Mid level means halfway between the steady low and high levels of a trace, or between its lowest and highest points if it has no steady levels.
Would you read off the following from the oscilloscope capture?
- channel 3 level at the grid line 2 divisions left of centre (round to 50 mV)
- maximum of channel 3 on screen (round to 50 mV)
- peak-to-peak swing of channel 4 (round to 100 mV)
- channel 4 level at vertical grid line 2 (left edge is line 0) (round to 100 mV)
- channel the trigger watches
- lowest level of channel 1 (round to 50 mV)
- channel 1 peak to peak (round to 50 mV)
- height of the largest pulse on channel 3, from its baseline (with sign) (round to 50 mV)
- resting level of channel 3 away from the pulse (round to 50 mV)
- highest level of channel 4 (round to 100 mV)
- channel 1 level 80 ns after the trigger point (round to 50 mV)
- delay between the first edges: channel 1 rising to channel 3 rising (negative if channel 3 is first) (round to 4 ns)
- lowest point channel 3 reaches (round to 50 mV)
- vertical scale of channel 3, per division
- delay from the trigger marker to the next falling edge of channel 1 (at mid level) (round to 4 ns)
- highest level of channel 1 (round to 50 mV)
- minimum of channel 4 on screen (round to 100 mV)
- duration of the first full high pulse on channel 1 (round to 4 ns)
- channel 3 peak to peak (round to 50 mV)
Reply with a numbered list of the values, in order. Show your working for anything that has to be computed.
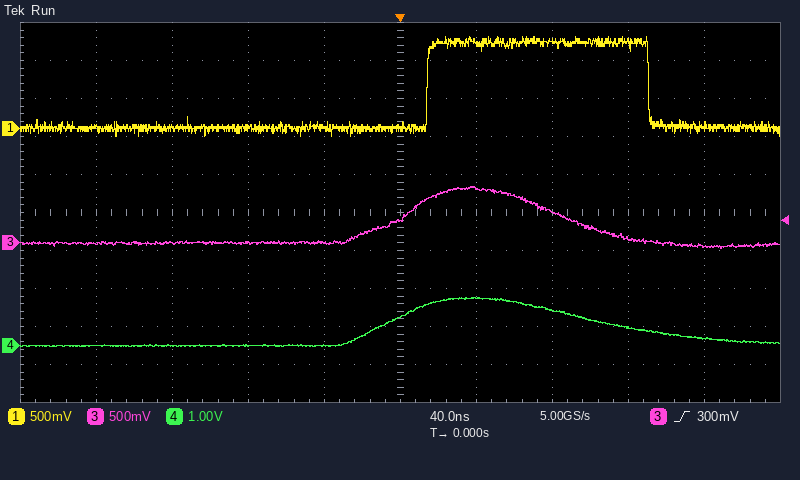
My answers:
1. 0 mV
2. 750 mV
3. 1.3 V − (0.0 V) = 1.3 V
4. 0.0 V
5. channel 3
6. -100 mV
7. 1.20 V − (-100 mV) = 1.30 V
8. 750 mV − (0 mV) = +750 mV
9. 0 mV
10. 1.3 V
11. 1.15 V
12. -12 ns
13. -50 mV
14. 500 mV
15. 132 ns
16. 1.20 V
17. 0.0 V
18. 116 ns
19. 750 mV − (-50 mV) = 800 mV
